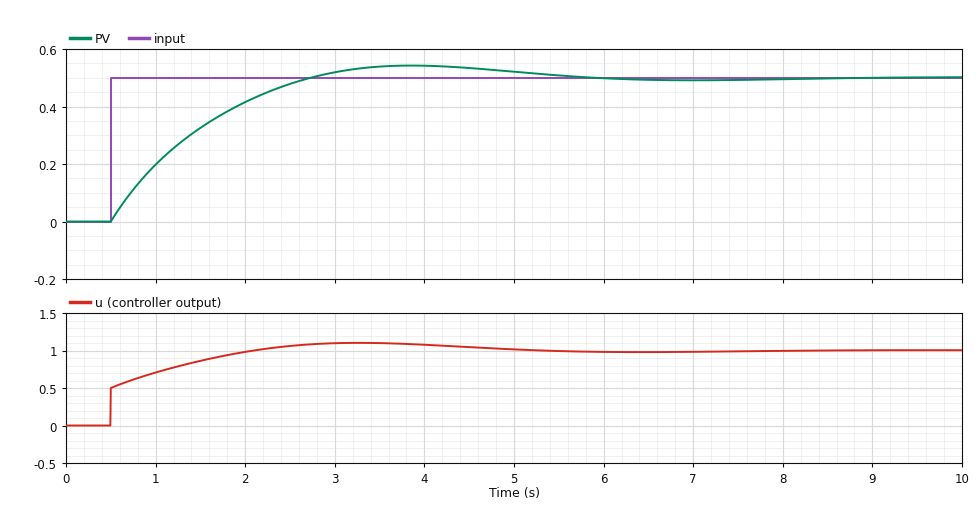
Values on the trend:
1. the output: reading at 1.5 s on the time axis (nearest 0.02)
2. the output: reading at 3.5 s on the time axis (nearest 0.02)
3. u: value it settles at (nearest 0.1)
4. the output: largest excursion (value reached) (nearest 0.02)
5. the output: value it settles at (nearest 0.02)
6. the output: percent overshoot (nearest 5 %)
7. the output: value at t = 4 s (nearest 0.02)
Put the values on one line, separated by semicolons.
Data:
0.32; 0.54; 1.0; 0.54; 0.50; 10 %; 0.54
